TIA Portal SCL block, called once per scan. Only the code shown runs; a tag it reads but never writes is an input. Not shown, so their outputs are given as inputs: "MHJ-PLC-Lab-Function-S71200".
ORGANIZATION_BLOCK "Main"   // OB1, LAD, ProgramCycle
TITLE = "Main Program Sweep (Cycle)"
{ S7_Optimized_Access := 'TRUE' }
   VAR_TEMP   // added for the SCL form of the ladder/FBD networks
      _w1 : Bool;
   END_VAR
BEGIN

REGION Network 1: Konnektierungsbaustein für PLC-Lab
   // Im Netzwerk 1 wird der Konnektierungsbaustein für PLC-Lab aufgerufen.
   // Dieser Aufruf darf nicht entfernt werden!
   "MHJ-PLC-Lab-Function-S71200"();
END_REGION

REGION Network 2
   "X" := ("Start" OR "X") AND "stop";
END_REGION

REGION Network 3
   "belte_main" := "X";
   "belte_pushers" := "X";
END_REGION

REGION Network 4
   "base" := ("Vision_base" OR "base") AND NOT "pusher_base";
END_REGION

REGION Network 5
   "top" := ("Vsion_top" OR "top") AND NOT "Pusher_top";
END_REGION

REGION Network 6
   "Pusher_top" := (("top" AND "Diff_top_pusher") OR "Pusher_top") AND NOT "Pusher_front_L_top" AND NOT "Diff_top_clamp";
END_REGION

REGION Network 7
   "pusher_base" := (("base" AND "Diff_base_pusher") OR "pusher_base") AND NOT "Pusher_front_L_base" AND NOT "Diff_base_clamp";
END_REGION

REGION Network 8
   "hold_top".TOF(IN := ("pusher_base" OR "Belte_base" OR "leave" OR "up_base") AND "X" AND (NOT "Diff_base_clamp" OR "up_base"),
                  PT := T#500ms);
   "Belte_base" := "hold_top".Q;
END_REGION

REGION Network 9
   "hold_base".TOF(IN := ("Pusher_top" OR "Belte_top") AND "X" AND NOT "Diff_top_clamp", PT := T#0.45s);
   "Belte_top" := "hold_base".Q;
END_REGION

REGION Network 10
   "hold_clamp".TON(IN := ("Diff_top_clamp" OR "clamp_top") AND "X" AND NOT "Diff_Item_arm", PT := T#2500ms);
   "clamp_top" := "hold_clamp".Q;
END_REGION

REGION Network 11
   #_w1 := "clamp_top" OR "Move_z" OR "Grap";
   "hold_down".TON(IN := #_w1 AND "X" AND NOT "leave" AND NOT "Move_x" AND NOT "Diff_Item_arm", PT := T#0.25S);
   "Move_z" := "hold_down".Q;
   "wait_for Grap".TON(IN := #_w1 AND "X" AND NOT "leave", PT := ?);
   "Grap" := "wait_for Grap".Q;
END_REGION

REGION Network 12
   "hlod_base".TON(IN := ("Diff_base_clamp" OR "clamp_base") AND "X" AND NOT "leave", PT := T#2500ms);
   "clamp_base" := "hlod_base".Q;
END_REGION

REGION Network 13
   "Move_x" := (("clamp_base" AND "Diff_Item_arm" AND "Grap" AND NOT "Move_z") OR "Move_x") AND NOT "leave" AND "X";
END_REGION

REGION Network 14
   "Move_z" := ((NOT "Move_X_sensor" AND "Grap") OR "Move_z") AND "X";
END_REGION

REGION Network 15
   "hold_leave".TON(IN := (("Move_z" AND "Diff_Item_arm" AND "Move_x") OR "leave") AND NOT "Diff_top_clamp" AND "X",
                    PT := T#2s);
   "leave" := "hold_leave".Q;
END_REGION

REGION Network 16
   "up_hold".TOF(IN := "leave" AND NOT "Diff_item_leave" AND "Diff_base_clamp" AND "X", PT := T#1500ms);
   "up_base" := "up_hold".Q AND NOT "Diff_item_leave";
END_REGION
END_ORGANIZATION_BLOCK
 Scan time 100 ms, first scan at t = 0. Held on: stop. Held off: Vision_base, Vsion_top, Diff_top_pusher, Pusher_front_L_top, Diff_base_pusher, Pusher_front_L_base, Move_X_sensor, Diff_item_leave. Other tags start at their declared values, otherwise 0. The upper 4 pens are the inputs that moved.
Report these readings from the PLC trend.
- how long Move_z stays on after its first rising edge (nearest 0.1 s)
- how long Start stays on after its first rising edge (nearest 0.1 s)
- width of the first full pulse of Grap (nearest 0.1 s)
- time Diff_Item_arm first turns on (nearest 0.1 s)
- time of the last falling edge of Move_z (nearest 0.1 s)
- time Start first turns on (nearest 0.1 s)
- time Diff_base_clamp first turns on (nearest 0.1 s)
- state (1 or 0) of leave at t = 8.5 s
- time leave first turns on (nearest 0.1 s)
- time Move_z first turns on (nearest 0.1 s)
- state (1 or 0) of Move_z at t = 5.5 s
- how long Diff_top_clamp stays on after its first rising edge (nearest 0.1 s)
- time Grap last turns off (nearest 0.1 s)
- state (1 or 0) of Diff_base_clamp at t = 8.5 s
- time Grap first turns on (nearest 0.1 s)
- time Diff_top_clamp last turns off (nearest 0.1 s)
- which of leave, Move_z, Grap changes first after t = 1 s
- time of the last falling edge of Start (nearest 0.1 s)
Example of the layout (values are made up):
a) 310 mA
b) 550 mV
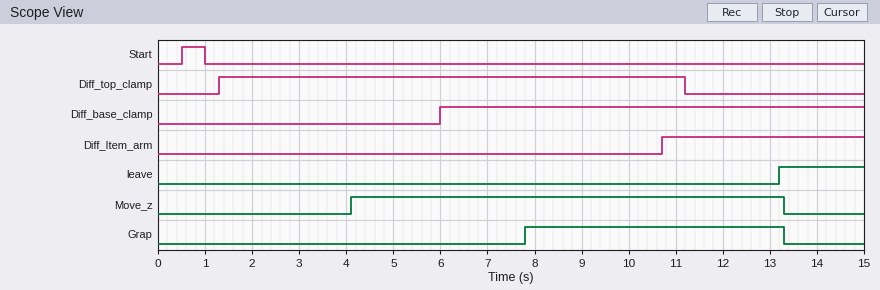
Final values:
a) 9.2 s
b) 0.5 s
c) 5.5 s
d) 10.7 s
e) 13.3 s
f) 0.5 s
g) 6.0 s
h) 0
i) 13.2 s
j) 4.1 s
k) 1
l) 9.9 s
m) 13.3 s
n) 1
o) 7.8 s
p) 11.2 s
q) Move_z
r) 1.0 s
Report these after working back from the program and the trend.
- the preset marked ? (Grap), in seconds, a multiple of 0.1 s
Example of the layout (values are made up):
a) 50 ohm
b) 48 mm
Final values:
a) 4.0 s
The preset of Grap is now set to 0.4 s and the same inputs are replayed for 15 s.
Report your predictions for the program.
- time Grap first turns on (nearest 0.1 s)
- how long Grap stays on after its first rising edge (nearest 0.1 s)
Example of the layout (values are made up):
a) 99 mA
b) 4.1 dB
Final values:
a) 4.2 s
b) 9.1 s
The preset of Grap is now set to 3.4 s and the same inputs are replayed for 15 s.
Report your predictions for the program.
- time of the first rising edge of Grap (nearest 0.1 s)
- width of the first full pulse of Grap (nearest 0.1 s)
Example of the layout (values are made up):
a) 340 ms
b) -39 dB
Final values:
a) 7.2 s
b) 6.1 s
